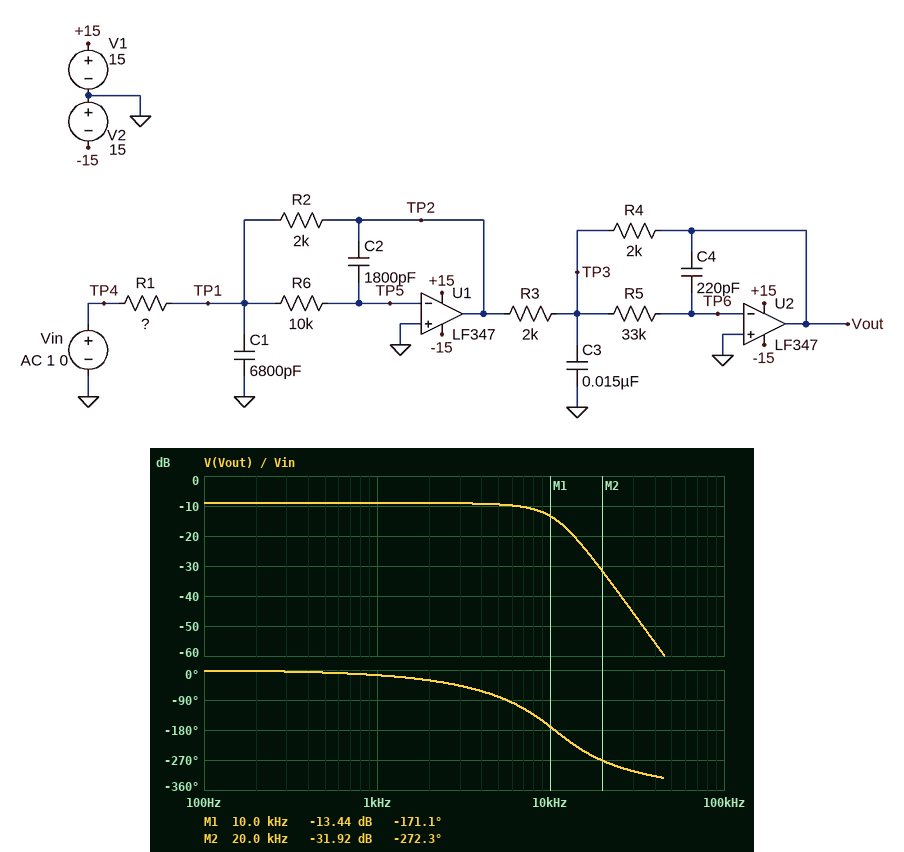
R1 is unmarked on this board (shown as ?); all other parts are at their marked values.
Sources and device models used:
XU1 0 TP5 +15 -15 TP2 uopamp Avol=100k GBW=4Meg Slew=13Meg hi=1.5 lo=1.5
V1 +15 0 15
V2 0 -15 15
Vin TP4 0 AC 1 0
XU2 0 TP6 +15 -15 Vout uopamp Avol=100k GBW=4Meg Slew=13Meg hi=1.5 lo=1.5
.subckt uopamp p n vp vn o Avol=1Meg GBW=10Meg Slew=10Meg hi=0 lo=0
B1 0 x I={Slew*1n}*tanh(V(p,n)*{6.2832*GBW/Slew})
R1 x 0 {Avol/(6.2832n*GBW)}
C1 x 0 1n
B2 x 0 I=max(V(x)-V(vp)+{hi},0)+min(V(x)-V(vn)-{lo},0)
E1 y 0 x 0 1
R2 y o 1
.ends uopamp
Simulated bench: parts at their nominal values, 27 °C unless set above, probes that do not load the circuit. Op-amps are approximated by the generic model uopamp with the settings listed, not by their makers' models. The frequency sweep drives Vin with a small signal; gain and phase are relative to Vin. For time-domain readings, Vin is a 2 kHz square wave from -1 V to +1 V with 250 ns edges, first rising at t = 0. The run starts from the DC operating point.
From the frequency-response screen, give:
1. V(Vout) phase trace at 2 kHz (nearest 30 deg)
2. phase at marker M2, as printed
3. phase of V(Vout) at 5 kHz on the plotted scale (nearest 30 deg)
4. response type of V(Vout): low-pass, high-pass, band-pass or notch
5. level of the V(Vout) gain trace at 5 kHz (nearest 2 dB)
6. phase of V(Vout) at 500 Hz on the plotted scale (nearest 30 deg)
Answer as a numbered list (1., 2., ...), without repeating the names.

1. -30 deg
2. -272.3 deg
3. -90 deg
4. low-pass
5. -10 dB
6. 0 deg
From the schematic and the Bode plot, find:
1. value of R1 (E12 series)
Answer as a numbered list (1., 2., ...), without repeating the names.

1. 5.6 kΩ
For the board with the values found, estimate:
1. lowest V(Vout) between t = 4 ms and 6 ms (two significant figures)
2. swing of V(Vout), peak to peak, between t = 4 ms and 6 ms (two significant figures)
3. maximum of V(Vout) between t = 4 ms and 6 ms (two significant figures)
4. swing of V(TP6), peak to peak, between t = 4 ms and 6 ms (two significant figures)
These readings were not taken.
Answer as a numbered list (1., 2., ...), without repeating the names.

1. -400 mV
2. 800 mV
3. 400 mV
4. 1.3 mV
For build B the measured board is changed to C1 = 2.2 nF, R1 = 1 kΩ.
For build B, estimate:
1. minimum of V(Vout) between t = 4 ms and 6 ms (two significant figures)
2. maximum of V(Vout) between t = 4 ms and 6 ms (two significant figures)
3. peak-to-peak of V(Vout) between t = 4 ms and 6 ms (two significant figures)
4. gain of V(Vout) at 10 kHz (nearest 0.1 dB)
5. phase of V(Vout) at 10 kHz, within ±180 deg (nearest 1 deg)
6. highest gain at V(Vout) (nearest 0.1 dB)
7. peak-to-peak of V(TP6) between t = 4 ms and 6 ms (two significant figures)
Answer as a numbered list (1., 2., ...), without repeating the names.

1. -1.9 V
2. 1.9 V
3. 3.9 V
4. -4.9 dB
5. -161 deg
6. 6.0 dB
7. 4.3 mV
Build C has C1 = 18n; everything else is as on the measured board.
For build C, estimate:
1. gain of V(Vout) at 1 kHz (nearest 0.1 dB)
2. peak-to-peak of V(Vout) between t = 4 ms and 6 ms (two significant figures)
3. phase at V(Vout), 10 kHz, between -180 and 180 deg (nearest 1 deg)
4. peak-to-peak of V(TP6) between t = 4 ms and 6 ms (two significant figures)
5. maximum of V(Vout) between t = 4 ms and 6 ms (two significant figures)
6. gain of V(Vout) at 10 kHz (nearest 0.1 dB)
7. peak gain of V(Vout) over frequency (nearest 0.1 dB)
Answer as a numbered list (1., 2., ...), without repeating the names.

1. -8.8 dB
2. 980 mV
3. 146 deg
4. 1.2 mV
5. 490 mV
6. -16.0 dB
7. -7.6 dB
